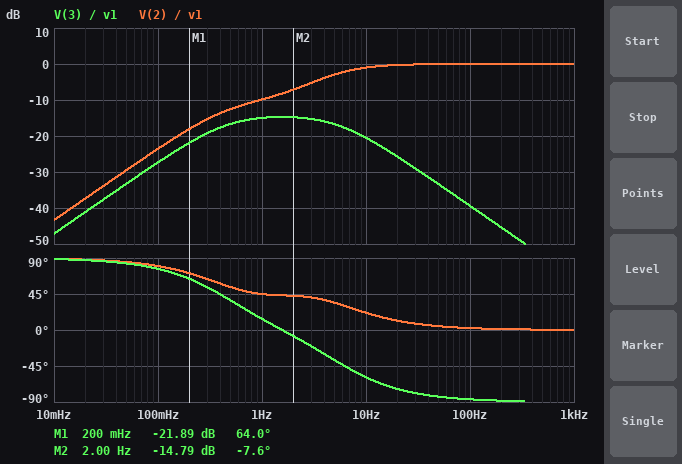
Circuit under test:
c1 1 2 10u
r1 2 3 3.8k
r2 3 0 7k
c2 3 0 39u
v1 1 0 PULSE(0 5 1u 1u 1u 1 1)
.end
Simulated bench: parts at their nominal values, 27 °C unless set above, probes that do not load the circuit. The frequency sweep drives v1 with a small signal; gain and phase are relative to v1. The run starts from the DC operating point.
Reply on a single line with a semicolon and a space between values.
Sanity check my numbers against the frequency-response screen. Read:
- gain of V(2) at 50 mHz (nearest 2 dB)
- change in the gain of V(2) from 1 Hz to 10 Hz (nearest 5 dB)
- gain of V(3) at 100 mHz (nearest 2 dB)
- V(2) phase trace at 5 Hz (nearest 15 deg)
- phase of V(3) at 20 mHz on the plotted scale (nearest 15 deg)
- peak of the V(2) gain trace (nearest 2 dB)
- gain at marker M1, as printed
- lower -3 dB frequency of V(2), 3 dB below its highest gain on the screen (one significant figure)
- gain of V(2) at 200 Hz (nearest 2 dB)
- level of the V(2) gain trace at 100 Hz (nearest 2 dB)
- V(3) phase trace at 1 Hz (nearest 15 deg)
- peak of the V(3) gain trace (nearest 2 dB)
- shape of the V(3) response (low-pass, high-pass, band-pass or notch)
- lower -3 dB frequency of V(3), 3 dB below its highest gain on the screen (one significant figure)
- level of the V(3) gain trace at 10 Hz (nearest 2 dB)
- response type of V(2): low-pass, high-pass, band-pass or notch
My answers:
-30 dB; 10 dB; -28 dB; 30 deg; 90 deg; 0 dB; -21.89 dB; 5 Hz; 0 dB; 0 dB; 15 deg; -14 dB; band-pass; 400 mHz; -20 dB; high-pass
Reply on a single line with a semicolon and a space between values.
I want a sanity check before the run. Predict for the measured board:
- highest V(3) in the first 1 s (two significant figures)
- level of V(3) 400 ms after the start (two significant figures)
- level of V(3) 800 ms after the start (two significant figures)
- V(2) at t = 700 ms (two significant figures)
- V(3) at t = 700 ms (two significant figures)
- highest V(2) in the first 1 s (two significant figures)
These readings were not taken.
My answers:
790 mV; 350 mV; 110 mV; 170 mV; 150 mV; 5.0 V
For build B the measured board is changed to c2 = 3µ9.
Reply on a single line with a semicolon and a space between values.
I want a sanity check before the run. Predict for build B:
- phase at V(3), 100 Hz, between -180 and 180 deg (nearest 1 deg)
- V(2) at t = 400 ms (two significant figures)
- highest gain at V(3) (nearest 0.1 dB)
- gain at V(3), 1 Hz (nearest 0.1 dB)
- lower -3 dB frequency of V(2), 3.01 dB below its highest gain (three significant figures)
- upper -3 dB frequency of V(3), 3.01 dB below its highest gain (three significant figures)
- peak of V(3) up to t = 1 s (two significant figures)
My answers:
-78 deg; 180 mV; -5.7 dB; -9.3 dB; 1.87 Hz; 21.9 Hz; 2.3 V
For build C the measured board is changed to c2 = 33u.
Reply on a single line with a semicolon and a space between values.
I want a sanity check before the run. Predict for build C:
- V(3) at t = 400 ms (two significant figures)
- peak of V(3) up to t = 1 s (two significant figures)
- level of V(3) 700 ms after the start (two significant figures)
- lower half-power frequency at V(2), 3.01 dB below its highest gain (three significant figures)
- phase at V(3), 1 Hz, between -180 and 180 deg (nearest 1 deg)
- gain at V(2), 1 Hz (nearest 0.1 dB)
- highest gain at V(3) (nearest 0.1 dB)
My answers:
340 mV; 890 mV; 130 mV; 4.97 Hz; 17 deg; -9.3 dB; -13.7 dB
